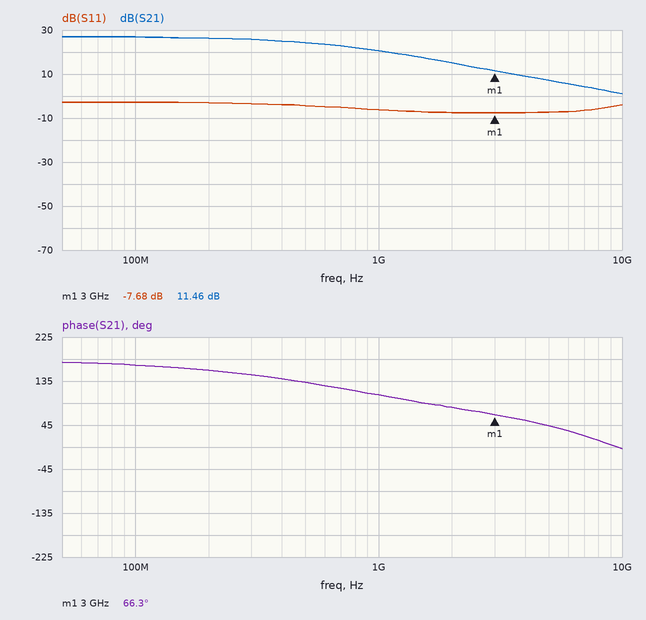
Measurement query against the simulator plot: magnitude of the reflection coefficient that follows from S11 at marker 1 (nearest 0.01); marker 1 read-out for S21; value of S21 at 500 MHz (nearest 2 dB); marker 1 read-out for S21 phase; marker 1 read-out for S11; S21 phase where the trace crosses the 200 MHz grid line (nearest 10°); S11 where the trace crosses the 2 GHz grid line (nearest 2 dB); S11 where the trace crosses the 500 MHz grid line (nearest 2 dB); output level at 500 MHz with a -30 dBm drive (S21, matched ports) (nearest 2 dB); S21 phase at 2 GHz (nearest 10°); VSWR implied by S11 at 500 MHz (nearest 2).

0.41
11.46 dB
24 dB
66.3°
-7.68 dB
160°
-8 dB
-4 dB
-6 dBm
80°
4
